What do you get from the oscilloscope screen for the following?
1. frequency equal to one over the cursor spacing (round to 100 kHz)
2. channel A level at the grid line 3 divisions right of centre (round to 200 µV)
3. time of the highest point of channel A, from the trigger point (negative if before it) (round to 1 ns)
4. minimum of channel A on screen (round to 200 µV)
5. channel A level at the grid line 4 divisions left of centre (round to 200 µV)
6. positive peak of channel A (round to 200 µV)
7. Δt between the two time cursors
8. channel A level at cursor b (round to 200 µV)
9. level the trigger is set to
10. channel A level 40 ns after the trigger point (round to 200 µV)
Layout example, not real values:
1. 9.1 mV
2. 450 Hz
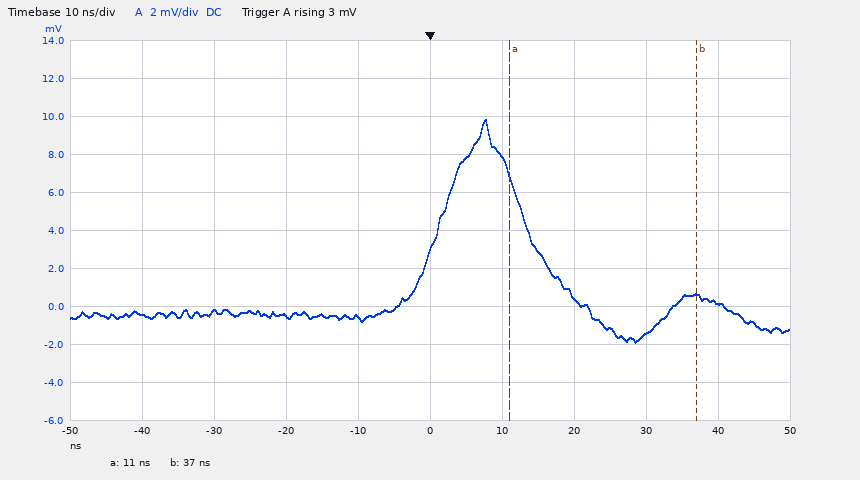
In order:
1. 38.5 MHz
2. -1.4 mV
3. +8 ns
4. -1.8 mV
5. -400 µV
6. 9.8 mV
7. 26 ns
8. 600 µV
9. 3 mV
10. 200 µV
